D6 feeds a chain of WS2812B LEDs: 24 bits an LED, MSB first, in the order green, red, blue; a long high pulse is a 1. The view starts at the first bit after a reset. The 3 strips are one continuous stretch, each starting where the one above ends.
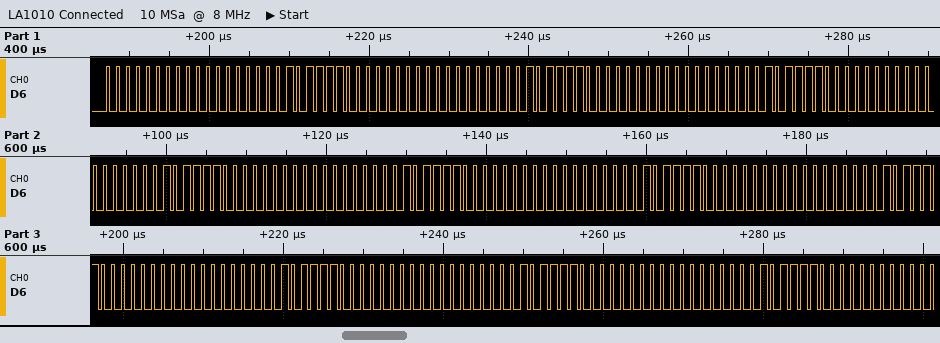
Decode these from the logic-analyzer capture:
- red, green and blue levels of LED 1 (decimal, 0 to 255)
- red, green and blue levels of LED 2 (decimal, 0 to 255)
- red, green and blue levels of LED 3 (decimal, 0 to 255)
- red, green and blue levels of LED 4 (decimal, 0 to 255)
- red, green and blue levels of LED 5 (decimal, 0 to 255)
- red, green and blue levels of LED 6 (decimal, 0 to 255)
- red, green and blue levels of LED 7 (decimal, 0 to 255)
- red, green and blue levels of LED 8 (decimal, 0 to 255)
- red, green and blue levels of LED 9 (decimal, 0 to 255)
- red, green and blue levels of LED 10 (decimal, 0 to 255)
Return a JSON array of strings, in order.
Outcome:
["0, 0, 47", "0, 0, 47", "0, 0, 47", "0, 0, 47", "0, 0, 47", "0, 0, 47", "0, 0, 47", "0, 0, 47", "0, 0, 47", "0, 0, 47"]
